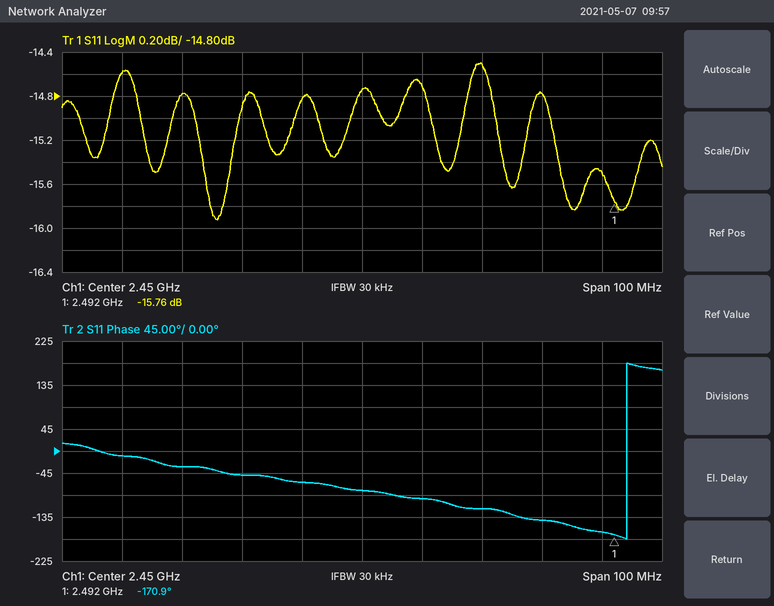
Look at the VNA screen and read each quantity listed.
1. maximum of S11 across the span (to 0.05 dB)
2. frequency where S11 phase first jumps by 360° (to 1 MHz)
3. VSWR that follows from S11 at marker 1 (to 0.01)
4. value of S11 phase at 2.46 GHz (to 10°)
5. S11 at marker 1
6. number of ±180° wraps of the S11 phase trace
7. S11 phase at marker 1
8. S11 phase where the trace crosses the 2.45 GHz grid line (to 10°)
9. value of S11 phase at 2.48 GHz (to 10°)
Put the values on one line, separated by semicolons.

-14.50 dB; 2.494 GHz; 1.39; -100°; -15.76 dB; 1; -170.9°; -80°; -140°
